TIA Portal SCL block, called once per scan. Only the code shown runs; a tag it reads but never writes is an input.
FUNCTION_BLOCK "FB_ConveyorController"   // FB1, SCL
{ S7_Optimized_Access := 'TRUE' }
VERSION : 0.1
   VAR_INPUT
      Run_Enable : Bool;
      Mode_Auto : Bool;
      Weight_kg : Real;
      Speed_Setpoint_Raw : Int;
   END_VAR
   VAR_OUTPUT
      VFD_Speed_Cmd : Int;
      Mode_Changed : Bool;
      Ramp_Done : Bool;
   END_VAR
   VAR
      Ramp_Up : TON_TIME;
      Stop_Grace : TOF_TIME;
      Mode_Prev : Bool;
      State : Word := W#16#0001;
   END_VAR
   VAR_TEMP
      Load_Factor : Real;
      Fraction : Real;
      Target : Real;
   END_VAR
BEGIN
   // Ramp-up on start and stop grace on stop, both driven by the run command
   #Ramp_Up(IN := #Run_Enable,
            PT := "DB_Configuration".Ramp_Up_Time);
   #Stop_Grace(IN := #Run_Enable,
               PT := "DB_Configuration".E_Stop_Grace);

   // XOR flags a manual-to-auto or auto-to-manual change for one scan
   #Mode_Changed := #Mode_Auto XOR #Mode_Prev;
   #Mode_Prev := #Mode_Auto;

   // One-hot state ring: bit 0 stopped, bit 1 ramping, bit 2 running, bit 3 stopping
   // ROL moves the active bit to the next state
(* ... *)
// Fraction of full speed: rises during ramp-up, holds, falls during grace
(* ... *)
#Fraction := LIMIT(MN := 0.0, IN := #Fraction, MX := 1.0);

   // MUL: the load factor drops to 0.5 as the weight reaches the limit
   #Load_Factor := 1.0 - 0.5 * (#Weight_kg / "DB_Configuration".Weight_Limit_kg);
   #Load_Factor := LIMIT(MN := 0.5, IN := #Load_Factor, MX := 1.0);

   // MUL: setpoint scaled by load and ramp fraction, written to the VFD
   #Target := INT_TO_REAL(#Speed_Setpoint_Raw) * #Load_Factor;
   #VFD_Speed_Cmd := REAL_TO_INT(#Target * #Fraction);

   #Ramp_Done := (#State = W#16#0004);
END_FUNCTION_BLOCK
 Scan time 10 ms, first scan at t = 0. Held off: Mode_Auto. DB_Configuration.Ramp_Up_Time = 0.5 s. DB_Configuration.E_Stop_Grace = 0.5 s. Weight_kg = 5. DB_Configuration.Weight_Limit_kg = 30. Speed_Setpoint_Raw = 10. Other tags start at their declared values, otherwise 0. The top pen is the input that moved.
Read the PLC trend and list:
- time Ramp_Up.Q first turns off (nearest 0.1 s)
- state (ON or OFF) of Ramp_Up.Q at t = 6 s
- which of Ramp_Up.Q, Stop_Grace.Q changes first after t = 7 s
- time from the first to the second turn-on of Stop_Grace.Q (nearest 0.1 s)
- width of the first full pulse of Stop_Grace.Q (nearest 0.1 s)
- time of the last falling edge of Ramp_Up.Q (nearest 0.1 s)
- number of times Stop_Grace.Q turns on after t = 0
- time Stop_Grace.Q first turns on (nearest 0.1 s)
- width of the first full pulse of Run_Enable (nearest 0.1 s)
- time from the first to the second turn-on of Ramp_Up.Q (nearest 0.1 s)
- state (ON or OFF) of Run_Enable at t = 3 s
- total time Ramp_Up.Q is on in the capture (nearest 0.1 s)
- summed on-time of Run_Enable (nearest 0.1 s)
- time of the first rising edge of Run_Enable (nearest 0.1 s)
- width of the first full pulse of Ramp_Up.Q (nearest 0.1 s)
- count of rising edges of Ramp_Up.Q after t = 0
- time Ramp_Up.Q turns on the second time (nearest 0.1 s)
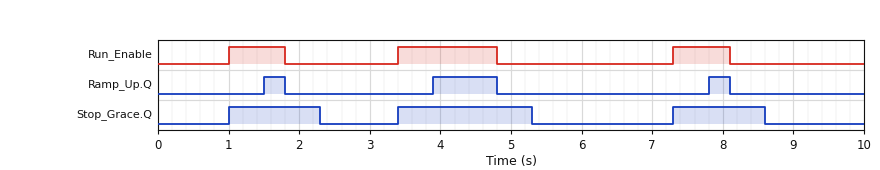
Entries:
1.8 s
OFF
Stop_Grace.Q
2.4 s
1.3 s
8.1 s
3
1.0 s
0.8 s
2.4 s
OFF
1.5 s
3.0 s
1.0 s
0.3 s
3
3.9 s
